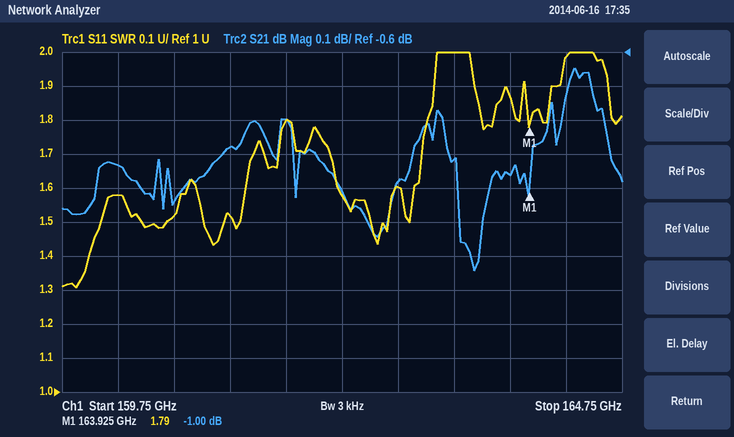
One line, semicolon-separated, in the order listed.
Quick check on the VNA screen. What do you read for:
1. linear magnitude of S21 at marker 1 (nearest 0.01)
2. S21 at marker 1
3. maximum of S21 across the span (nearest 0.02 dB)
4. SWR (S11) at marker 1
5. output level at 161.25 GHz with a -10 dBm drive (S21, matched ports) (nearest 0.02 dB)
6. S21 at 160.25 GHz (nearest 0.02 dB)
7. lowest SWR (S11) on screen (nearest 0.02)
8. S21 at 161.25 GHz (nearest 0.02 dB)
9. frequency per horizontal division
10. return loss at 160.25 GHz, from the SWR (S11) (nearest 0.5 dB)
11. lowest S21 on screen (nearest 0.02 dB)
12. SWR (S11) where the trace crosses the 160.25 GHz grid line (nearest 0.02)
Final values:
0.89; -1.00 dB; -0.64 dB; 1.79; -10.88 dBm; -0.94 dB; 1.30; -0.88 dB; 500 MHz; 13.0 dB; -1.24 dB; 1.58
